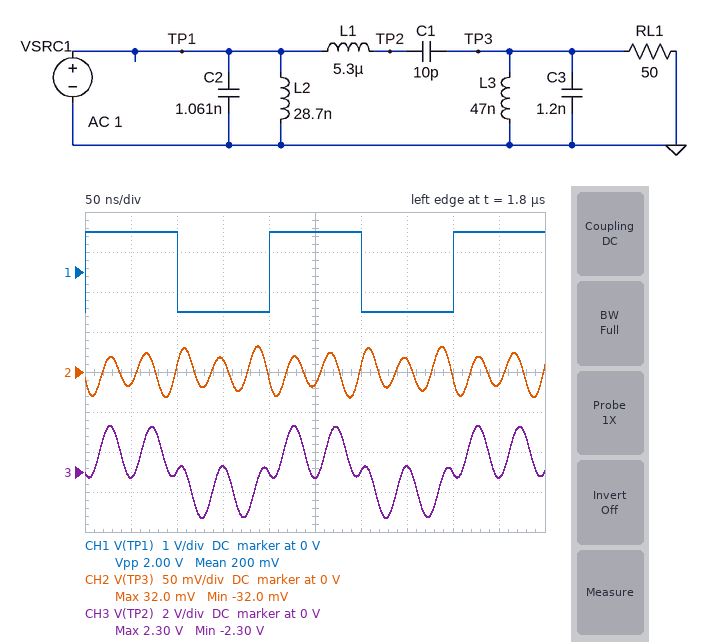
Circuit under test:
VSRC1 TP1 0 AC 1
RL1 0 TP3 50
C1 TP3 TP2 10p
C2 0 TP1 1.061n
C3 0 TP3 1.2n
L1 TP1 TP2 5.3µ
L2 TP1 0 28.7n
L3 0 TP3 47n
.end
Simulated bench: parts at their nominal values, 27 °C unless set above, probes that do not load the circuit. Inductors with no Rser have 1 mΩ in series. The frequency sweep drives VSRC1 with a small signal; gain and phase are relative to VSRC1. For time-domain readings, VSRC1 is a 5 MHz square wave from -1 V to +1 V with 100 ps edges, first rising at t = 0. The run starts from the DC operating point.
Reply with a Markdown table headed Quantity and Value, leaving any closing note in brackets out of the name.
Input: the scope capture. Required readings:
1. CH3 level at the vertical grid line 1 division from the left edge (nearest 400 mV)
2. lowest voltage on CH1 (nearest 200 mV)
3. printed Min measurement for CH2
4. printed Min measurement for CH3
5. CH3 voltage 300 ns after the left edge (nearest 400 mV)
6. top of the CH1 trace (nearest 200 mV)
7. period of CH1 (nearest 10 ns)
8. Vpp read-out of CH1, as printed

| Quantity | Value |
|---|---|
| CH3 level at the vertical grid line 1 division from the left edge | -400 mV |
| lowest voltage on CH1 | -1.0 V |
| printed Min measurement for CH2 | -32.0 mV |
| printed Min measurement for CH3 | -2.30 V |
| CH3 voltage 300 ns after the left edge | 0 V |
| top of the CH1 trace | 1.0 V |
| period of CH1 | 200 ns |
| Vpp read-out of CH1, as printed | 2.00 V |
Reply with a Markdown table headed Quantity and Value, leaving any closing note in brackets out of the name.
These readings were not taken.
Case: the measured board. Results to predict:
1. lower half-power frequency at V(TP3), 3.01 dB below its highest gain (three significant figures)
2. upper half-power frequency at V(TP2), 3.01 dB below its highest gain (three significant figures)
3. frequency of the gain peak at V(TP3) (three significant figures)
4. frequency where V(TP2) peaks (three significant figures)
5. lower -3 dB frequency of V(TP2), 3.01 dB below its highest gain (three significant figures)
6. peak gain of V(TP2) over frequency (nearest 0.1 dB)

| Quantity | Value |
|---|---|
| lower half-power frequency at V(TP3), 3.01 dB below its highest gain | 21.7 MHz |
| upper half-power frequency at V(TP2), 3.01 dB below its highest gain | 22.8 MHz |
| frequency of the gain peak at V(TP3) | 22.3 MHz |
| frequency where V(TP2) peaks | 22.4 MHz |
| lower -3 dB frequency of V(TP2), 3.01 dB below its highest gain | 21.9 MHz |
| peak gain of V(TP2) over frequency | 27.8 dB |
